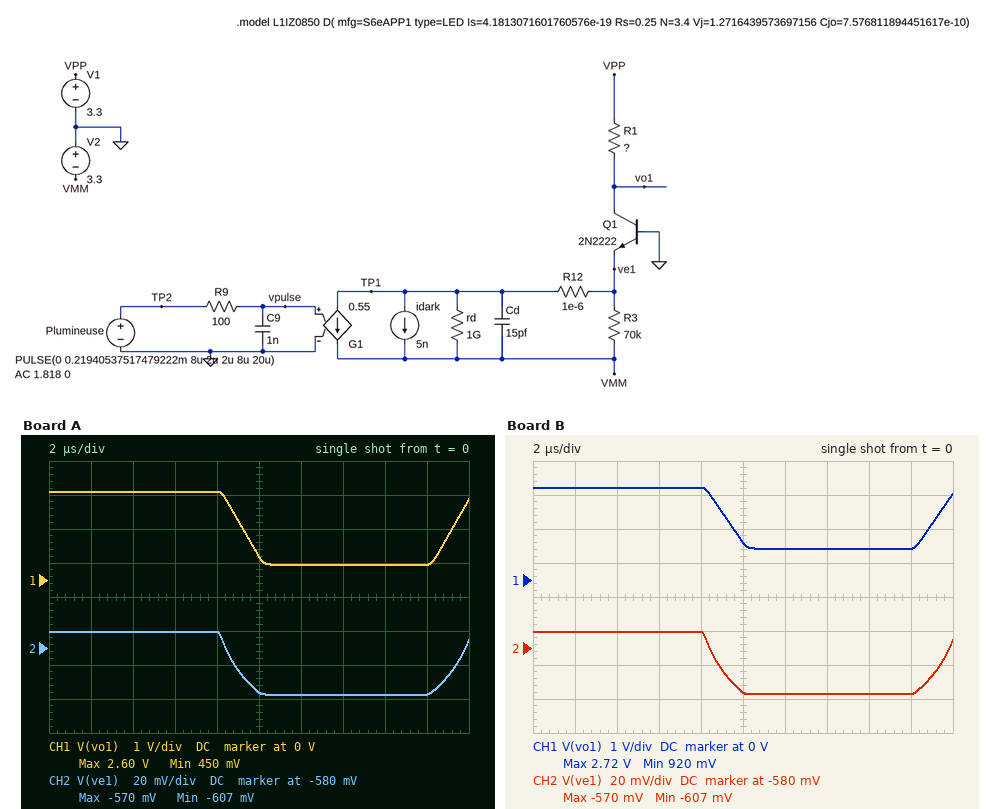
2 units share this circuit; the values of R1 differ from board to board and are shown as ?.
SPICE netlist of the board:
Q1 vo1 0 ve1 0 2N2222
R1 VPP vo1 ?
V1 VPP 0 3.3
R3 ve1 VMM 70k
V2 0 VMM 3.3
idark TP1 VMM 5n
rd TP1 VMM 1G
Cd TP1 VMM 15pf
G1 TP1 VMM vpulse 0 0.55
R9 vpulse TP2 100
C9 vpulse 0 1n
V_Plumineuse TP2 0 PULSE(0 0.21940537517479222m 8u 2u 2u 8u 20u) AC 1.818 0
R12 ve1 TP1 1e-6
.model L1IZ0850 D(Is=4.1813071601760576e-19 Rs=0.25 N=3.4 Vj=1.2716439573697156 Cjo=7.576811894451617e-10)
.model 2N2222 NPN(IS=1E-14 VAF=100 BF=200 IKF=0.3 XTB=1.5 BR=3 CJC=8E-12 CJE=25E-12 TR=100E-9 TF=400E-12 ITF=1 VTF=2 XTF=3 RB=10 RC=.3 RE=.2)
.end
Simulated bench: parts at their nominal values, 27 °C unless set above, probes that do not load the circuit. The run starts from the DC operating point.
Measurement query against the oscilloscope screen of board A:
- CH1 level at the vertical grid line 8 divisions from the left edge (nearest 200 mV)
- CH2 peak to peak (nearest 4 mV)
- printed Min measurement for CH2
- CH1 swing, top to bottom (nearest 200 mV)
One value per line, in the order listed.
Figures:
400 mV
36 mV
-607 mV
2.2 V
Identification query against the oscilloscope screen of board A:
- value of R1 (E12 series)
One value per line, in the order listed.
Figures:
18 kΩ
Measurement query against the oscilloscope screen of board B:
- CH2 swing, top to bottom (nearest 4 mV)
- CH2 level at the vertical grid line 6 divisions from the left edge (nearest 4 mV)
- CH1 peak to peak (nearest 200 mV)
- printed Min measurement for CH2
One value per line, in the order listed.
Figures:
36 mV
-608 mV
1.8 V
-607 mV
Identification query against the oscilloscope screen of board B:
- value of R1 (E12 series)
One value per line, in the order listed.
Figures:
15 kΩ
